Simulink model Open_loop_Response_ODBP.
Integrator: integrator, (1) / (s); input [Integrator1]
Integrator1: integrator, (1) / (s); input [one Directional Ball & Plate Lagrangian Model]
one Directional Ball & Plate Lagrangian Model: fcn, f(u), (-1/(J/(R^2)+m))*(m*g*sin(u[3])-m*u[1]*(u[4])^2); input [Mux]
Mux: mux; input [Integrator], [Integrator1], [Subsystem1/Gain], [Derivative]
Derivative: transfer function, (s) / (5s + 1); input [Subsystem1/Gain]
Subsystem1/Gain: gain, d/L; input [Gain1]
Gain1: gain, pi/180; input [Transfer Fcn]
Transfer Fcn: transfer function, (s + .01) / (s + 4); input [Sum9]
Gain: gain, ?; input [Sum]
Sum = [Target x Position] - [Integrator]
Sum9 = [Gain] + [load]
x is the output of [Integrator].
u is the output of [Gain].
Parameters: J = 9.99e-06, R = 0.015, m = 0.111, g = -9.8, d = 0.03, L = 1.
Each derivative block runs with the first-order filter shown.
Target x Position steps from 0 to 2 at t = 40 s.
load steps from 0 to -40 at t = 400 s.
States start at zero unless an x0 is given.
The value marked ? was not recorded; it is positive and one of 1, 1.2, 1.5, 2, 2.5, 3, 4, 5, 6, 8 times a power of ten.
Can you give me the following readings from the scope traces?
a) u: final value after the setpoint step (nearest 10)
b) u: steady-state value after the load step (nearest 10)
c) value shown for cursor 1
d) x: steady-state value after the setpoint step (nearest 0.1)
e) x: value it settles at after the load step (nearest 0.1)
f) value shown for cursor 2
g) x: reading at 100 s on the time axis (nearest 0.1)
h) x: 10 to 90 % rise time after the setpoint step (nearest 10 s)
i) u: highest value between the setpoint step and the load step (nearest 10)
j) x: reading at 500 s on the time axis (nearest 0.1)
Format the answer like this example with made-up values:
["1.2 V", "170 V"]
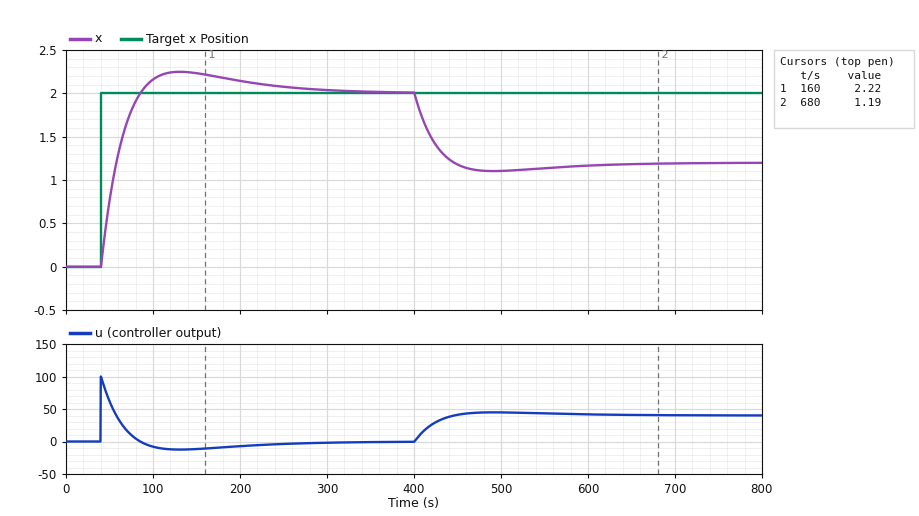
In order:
["0", "40", "2.22", "2.0", "1.2", "1.19", "2.2", "30 s", "100", "1.1"]
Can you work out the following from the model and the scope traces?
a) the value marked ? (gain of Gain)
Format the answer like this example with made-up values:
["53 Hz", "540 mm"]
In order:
["50"]
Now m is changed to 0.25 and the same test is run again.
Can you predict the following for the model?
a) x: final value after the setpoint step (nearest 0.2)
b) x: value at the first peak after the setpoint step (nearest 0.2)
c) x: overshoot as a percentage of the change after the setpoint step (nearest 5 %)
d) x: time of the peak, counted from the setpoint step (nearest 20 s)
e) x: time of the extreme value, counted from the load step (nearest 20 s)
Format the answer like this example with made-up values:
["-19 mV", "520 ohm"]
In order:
["2.0", "2.2", "10 %", "80 s", "80 s"]
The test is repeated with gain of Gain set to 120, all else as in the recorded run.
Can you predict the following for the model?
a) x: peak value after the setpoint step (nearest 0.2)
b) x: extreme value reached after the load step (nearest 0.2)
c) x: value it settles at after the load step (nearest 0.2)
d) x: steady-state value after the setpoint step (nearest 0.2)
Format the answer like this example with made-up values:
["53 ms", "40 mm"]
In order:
["2.2", "1.6", "1.6", "2.0"]
